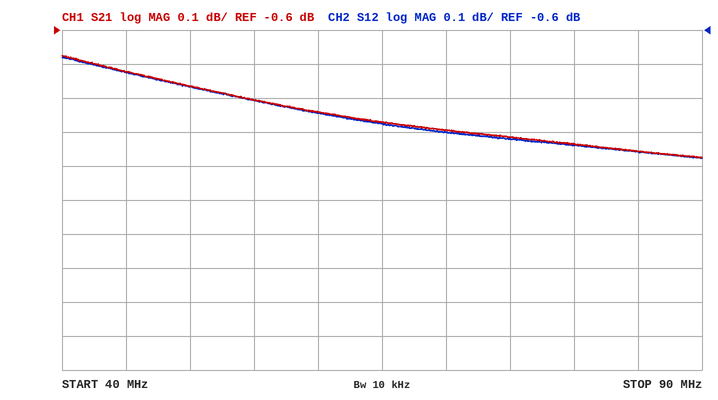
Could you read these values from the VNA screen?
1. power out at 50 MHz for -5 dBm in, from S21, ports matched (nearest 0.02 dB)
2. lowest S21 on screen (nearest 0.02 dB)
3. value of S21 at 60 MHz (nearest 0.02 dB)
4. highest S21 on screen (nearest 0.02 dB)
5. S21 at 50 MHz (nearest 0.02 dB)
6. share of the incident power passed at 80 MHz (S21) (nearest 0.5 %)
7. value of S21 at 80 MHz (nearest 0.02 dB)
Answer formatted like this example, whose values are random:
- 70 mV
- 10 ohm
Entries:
- -5.76 dBm
- -0.98 dB
- -0.84 dB
- -0.68 dB
- -0.76 dB
- 80.5 %
- -0.94 dB
